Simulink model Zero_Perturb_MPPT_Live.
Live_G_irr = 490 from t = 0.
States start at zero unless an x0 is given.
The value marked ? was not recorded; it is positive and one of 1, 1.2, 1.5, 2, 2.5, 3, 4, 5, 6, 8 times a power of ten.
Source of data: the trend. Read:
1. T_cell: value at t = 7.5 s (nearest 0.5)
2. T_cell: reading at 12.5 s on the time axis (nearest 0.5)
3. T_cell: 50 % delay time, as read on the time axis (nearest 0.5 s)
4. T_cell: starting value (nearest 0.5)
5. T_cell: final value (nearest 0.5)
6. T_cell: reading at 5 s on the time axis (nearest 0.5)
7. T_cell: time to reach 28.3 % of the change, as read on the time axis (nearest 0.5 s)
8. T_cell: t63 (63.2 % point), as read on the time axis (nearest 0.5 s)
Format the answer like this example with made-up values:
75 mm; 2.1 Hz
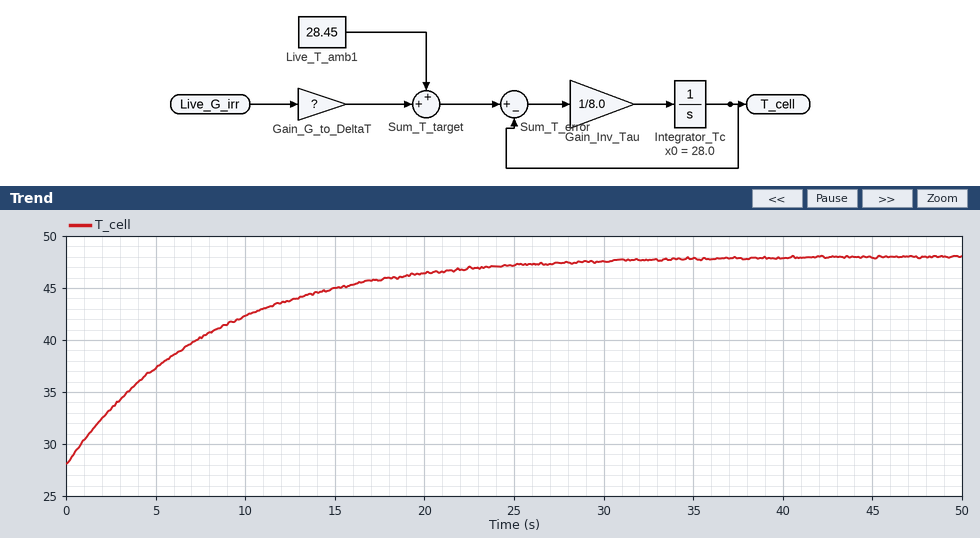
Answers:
40.0; 44.0; 5.5 s; 28.0; 48.0; 37.5; 2.5 s; 8.0 s
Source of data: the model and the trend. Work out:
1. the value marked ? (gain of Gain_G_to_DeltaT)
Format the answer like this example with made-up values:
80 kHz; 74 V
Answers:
0.04
